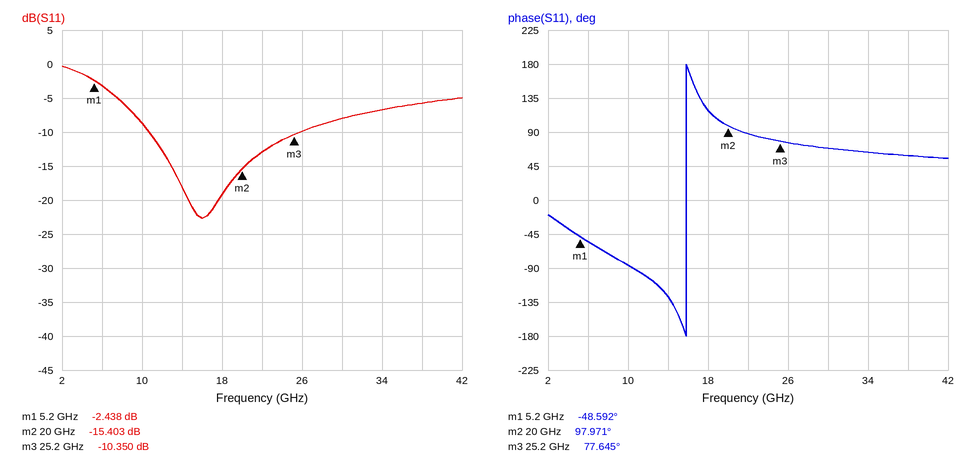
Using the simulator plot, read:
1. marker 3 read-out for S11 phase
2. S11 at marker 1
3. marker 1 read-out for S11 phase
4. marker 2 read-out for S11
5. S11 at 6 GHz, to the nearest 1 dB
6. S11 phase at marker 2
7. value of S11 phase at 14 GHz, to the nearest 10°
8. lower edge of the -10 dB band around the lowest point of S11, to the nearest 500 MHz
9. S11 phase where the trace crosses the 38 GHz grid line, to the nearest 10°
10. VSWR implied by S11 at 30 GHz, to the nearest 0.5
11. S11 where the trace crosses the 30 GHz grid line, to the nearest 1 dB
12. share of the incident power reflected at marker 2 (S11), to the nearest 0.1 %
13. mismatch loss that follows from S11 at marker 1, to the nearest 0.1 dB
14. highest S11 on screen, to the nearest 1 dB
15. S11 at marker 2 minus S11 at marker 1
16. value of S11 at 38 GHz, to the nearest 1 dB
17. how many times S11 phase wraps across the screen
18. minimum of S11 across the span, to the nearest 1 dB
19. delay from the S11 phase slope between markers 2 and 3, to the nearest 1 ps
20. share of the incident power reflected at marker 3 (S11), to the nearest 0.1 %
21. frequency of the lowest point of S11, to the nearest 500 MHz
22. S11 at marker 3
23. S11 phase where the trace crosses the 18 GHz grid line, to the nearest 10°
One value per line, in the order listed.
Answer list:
77.645°
-2.438 dB
-48.592°
-15.403 dB
-3 dB
97.971°
-130°
10.5 GHz
60°
2.5
-8 dB
2.9 %
3.7 dB
0 dB
-12.965 dB
-6 dB
1
-23 dB
11 ps
9.2 %
16.0 GHz
-10.350 dB
120°
